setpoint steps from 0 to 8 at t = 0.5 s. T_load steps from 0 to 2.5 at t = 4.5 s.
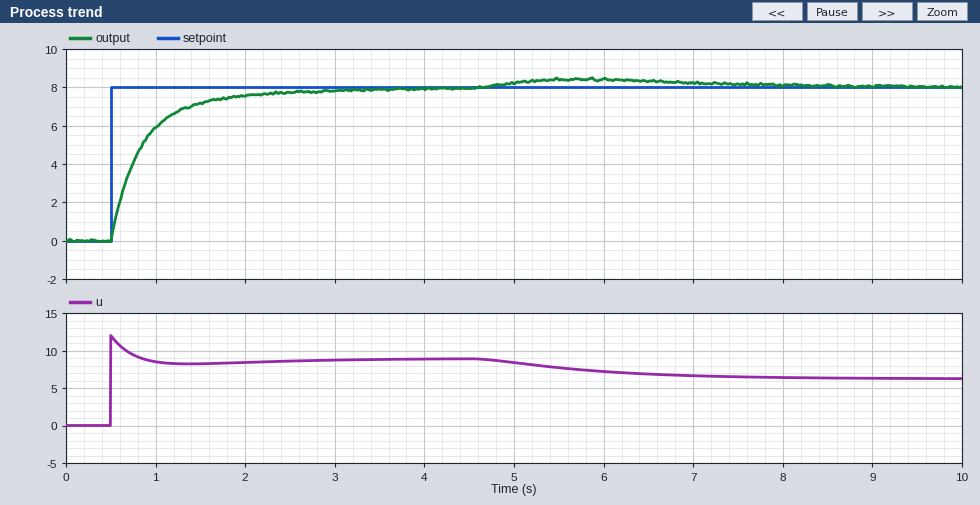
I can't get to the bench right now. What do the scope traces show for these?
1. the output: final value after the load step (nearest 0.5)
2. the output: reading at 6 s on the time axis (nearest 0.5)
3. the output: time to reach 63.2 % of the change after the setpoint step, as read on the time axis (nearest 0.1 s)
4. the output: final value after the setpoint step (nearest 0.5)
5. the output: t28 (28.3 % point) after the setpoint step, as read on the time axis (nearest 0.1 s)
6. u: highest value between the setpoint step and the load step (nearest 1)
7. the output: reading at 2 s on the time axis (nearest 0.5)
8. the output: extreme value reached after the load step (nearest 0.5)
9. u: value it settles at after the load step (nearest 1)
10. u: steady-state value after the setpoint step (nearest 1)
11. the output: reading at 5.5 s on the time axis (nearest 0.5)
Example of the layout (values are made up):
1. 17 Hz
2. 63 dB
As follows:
1. 8.0
2. 8.5
3. 0.9 s
4. 8.0
5. 0.6 s
6. 12
7. 7.5
8. 8.5
9. 6
10. 9
11. 8.5
